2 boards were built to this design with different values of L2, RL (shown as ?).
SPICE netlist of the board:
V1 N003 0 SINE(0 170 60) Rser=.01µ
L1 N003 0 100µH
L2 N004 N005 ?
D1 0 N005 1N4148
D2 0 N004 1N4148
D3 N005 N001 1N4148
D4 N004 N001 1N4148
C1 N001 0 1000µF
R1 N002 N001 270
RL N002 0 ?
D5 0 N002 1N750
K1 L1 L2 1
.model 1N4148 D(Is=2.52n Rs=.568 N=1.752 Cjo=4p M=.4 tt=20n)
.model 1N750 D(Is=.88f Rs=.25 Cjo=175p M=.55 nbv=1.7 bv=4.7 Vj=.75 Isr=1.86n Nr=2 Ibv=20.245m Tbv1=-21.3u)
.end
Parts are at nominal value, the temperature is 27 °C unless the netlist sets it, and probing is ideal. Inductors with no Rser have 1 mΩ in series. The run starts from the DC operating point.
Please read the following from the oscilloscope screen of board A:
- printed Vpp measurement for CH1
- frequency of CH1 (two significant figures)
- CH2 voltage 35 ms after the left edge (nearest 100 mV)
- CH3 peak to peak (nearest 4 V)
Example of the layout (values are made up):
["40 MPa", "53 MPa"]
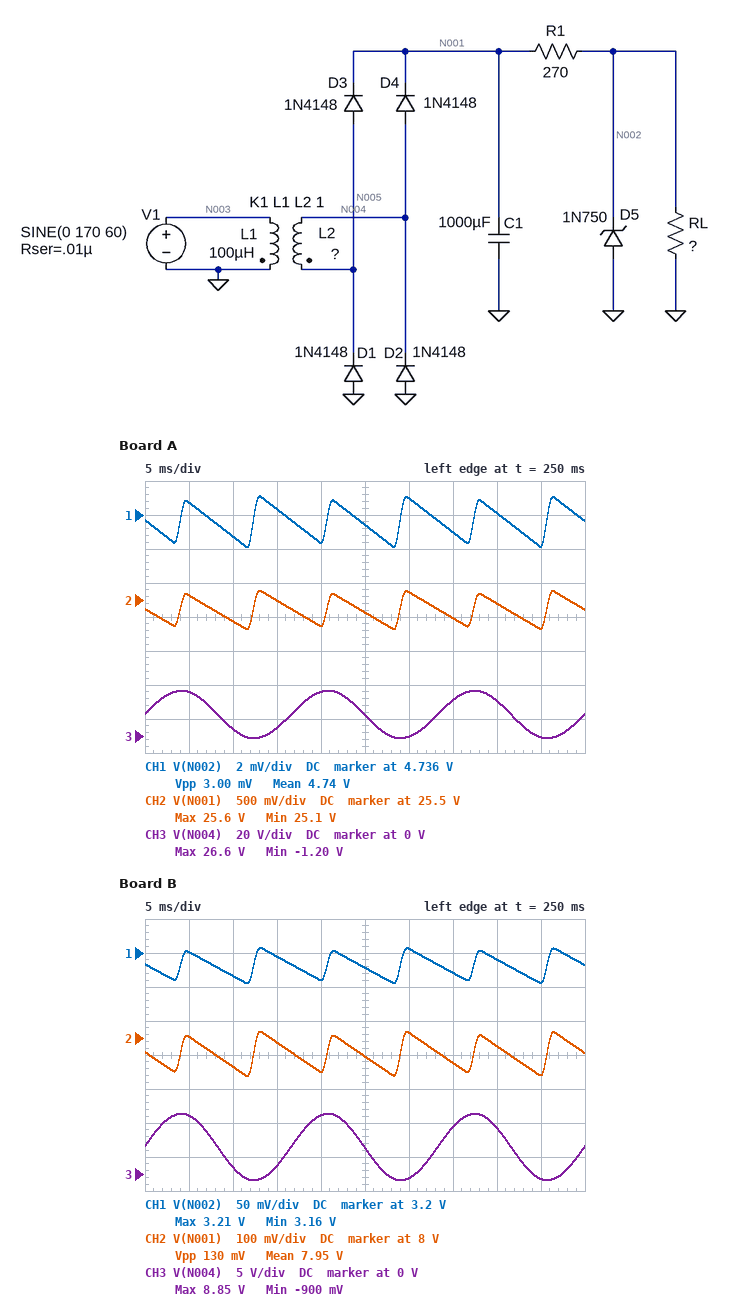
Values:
["3.00 mV", "120 Hz", "25.2 V", "28 V"]
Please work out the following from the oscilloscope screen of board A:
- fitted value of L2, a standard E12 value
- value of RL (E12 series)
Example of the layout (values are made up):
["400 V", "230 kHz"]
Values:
["2.7 µH", "120 Ω"]
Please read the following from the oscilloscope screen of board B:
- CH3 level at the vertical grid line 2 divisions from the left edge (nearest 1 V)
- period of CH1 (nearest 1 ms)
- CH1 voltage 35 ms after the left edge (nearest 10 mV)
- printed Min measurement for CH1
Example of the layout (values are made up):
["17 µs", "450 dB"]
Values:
["1 V", "8 ms", "3.17 V", "3.16 V"]
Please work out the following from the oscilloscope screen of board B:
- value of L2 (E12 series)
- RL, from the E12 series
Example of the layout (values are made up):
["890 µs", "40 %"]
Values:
["330 nH", "180 Ω"]
